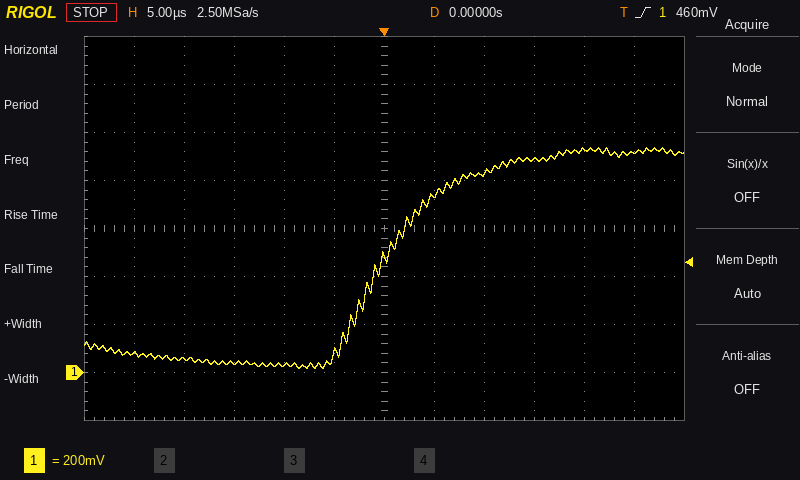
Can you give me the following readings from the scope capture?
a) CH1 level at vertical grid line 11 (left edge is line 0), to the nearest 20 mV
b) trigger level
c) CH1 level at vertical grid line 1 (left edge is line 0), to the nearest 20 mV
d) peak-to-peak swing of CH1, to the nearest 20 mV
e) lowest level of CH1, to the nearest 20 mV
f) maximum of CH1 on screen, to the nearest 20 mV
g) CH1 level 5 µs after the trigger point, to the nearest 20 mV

920 mV
460 mV
80 mV
920 mV
20 mV
940 mV
740 mV
